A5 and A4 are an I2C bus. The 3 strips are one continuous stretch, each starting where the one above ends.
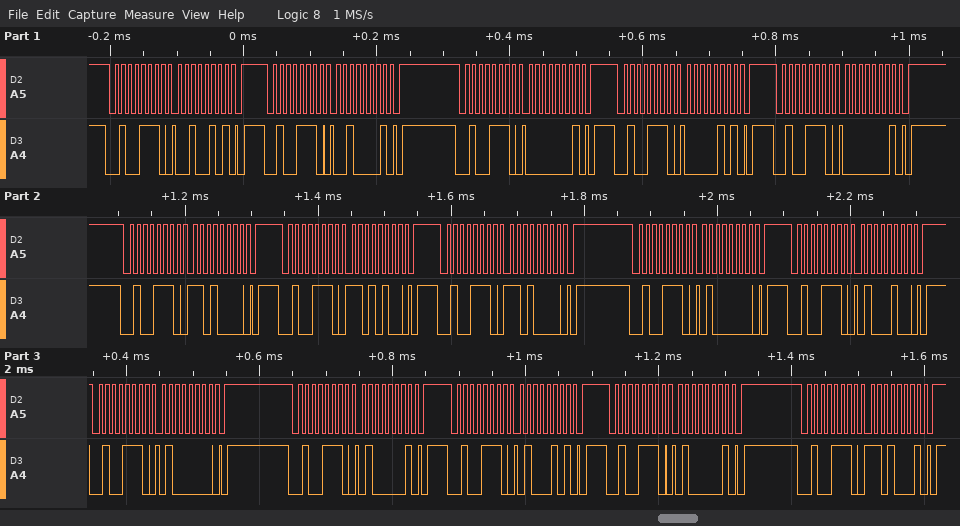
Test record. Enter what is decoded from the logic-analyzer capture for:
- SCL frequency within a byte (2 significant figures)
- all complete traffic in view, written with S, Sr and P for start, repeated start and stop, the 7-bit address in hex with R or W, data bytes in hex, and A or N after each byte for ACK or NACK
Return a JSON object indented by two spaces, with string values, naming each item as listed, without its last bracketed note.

{
  "SCL frequency within a byte": "100 kHz",
  "all complete traffic in view, written with S, Sr and P for start, repeated start and stop, the 7-bit address in hex with R or W, data bytes in hex, and A or N after each byte for ACK or NACK": "S 27W A 25 A P S 27W A 21 A P S 27W A 01 A P S 27W A 05 A P S 27W A 01 A P S 27W A D0 A P S 27W A D4 A P S 27W A D0 A P S 27W A 40 A P S 27W A 44 A P S 27W A 40 A P S 27W A 41 A P S 27W A 45 A P S 27W A 41 A P S 27W A D1 A P"
}
